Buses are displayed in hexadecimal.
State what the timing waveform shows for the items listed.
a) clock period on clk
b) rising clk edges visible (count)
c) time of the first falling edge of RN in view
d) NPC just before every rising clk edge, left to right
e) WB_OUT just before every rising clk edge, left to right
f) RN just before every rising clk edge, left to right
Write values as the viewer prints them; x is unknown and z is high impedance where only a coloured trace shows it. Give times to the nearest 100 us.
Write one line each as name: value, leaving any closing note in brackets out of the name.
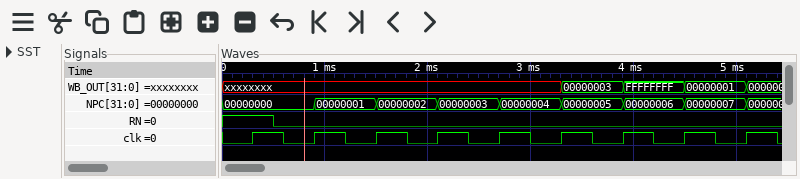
clock period on clk: 600 us
rising clk edges visible: 9
time of the first falling edge of RN in view: 500 us
NPC just before every rising clk edge, left to right: 00000000, 00000000, 00000001, 00000002, 00000003, 00000004, 00000005, 00000006, 00000007
WB_OUT just before every rising clk edge, left to right: xxxxxxxx, xxxxxxxx, xxxxxxxx, xxxxxxxx, xxxxxxxx, xxxxxxxx, 00000003, FFFFFFFF, 00000001
RN just before every rising clk edge, left to right: 1 0 0 0 0 0 0 0 0
